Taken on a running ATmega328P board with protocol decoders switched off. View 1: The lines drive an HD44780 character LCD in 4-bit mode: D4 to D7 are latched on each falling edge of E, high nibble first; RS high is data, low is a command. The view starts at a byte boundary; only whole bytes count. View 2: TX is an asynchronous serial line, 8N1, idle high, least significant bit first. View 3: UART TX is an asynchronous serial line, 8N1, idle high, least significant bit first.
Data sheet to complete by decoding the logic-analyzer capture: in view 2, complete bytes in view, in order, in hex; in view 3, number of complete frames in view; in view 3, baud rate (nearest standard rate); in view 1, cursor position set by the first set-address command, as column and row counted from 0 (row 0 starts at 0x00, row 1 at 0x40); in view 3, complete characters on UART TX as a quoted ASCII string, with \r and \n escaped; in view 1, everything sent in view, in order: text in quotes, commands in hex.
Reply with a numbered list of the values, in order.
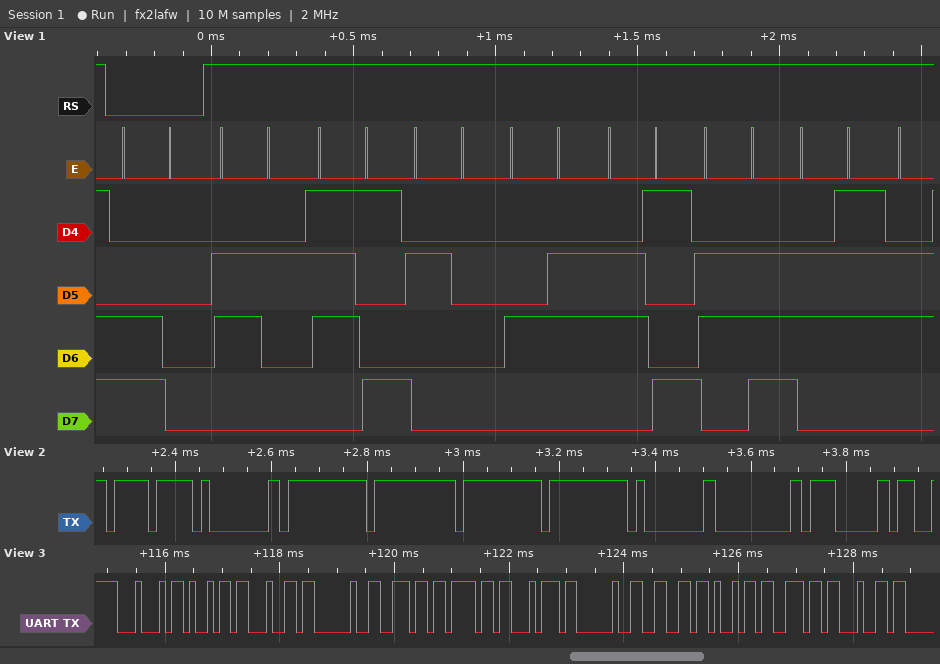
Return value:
1. EF 01 FF FF FF FF 01 00 07
2. 12
3. 9600 baud
4. column 0, row 1
5. "Did not find"
6. 0xC0 "by Fing"
